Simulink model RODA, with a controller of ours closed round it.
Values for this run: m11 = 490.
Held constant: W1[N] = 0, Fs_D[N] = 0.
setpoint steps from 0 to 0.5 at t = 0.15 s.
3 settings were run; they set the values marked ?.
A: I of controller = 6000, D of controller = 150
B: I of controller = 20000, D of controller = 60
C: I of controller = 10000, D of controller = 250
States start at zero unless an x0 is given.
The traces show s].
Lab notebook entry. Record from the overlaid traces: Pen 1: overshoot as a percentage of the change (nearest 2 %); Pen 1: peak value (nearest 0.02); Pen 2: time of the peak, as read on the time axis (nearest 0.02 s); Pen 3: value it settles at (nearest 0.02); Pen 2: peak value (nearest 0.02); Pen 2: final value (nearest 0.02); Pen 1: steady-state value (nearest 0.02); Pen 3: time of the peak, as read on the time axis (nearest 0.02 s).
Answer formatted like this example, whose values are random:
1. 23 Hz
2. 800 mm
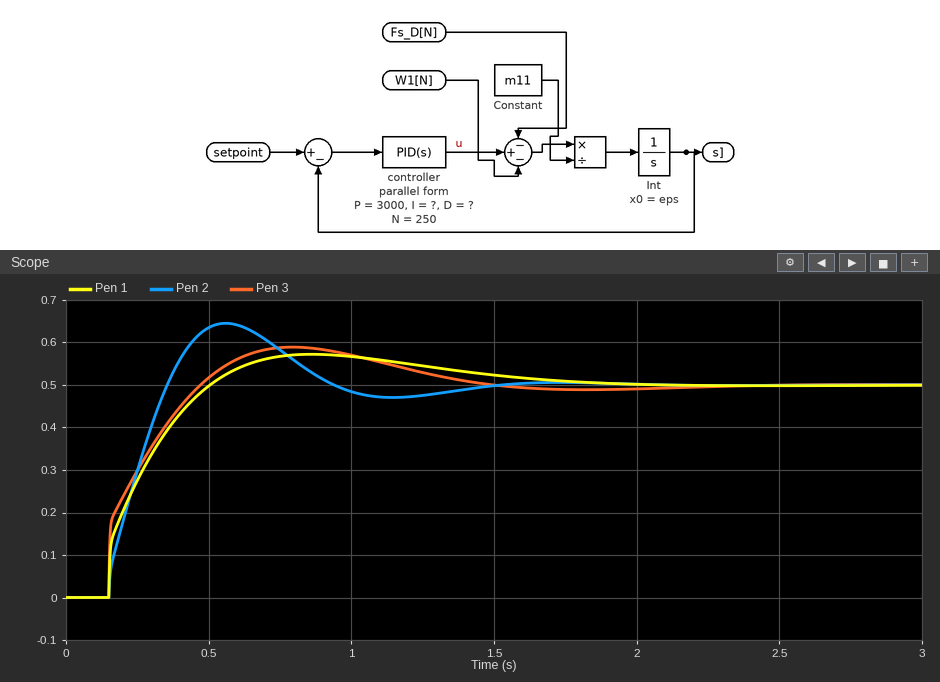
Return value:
1. 14 %
2. 0.58
3. 0.56 s
4. 0.50
5. 0.64
6. 0.50
7. 0.50
8. 0.80 s
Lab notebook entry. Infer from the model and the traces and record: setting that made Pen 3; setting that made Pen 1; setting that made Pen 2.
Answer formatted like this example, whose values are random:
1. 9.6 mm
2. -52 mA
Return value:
1. C
2. A
3. B
